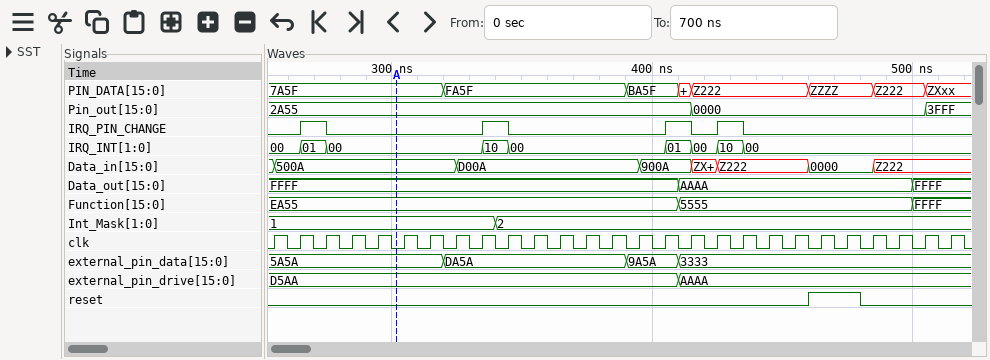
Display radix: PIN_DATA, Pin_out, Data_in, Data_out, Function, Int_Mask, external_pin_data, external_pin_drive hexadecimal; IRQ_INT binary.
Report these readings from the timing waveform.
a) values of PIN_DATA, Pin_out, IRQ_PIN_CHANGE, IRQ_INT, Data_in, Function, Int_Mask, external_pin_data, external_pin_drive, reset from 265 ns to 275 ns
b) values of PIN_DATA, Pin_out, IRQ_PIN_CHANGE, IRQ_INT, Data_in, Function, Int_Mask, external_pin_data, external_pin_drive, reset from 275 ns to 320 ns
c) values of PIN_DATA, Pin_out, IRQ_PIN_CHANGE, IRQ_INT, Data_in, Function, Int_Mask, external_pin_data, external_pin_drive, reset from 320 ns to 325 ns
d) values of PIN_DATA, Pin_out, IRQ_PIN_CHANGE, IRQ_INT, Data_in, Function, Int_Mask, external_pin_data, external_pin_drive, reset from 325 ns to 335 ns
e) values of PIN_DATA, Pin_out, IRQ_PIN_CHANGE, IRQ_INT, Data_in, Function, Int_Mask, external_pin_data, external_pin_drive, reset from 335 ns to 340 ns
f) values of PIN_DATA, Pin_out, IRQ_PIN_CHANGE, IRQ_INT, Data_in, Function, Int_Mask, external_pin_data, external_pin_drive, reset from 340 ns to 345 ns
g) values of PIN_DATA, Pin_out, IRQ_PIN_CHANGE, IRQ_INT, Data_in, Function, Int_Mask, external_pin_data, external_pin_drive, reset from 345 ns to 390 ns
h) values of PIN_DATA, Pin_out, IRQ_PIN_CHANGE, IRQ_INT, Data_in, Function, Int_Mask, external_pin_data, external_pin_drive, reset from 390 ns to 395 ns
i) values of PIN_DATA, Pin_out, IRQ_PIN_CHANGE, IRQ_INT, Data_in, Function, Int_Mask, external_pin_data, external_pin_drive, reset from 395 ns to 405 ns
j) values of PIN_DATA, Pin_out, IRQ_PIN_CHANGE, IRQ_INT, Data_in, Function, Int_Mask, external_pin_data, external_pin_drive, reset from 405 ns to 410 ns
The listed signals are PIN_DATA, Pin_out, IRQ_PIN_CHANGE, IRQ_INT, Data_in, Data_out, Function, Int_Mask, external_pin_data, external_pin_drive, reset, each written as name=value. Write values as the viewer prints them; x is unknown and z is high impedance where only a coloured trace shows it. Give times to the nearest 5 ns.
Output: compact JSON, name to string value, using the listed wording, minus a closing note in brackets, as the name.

{"values of PIN_DATA, Pin_out, IRQ_PIN_CHANGE, IRQ_INT, Data_in, Function, Int_Mask, external_pin_data, external_pin_drive, reset from 265 ns to 275 ns": "PIN_DATA=7A5F, Pin_out=2A55, IRQ_PIN_CHANGE=1, IRQ_INT=01, Data_in=500A, Function=EA55, Int_Mask=1, external_pin_data=5A5A, external_pin_drive=D5AA, reset=0", "values of PIN_DATA, Pin_out, IRQ_PIN_CHANGE, IRQ_INT, Data_in, Function, Int_Mask, external_pin_data, external_pin_drive, reset from 275 ns to 320 ns": "PIN_DATA=7A5F, Pin_out=2A55, IRQ_PIN_CHANGE=0, IRQ_INT=00, Data_in=500A, Function=EA55, Int_Mask=1, external_pin_data=5A5A, external_pin_drive=D5AA, reset=0", "values of PIN_DATA, Pin_out, IRQ_PIN_CHANGE, IRQ_INT, Data_in, Function, Int_Mask, external_pin_data, external_pin_drive, reset from 320 ns to 325 ns": "PIN_DATA=FA5F, Pin_out=2A55, IRQ_PIN_CHANGE=0, IRQ_INT=00, Data_in=500A, Function=EA55, Int_Mask=1, external_pin_data=DA5A, external_pin_drive=D5AA, reset=0", "values of PIN_DATA, Pin_out, IRQ_PIN_CHANGE, IRQ_INT, Data_in, Function, Int_Mask, external_pin_data, external_pin_drive, reset from 325 ns to 335 ns": "PIN_DATA=FA5F, Pin_out=2A55, IRQ_PIN_CHANGE=0, IRQ_INT=00, Data_in=D00A, Function=EA55, Int_Mask=1, external_pin_data=DA5A, external_pin_drive=D5AA, reset=0", "values of PIN_DATA, Pin_out, IRQ_PIN_CHANGE, IRQ_INT, Data_in, Function, Int_Mask, external_pin_data, external_pin_drive, reset from 335 ns to 340 ns": "PIN_DATA=FA5F, Pin_out=2A55, IRQ_PIN_CHANGE=1, IRQ_INT=10, Data_in=D00A, Function=EA55, Int_Mask=1, external_pin_data=DA5A, external_pin_drive=D5AA, reset=0", "values of PIN_DATA, Pin_out, IRQ_PIN_CHANGE, IRQ_INT, Data_in, Function, Int_Mask, external_pin_data, external_pin_drive, reset from 340 ns to 345 ns": "PIN_DATA=FA5F, Pin_out=2A55, IRQ_PIN_CHANGE=1, IRQ_INT=10, Data_in=D00A, Function=EA55, Int_Mask=2, external_pin_data=DA5A, external_pin_drive=D5AA, reset=0", "values of PIN_DATA, Pin_out, IRQ_PIN_CHANGE, IRQ_INT, Data_in, Function, Int_Mask, external_pin_data, external_pin_drive, reset from 345 ns to 390 ns": "PIN_DATA=FA5F, Pin_out=2A55, IRQ_PIN_CHANGE=0, IRQ_INT=00, Data_in=D00A, Function=EA55, Int_Mask=2, external_pin_data=DA5A, external_pin_drive=D5AA, reset=0", "values of PIN_DATA, Pin_out, IRQ_PIN_CHANGE, IRQ_INT, Data_in, Function, Int_Mask, external_pin_data, external_pin_drive, reset from 390 ns to 395 ns": "PIN_DATA=BA5F, Pin_out=2A55, IRQ_PIN_CHANGE=0, IRQ_INT=00, Data_in=D00A, Function=EA55, Int_Mask=2, external_pin_data=9A5A, external_pin_drive=D5AA, reset=0", "values of PIN_DATA, Pin_out, IRQ_PIN_CHANGE, IRQ_INT, Data_in, Function, Int_Mask, external_pin_data, external_pin_drive, reset from 395 ns to 405 ns": "PIN_DATA=BA5F, Pin_out=2A55, IRQ_PIN_CHANGE=0, IRQ_INT=00, Data_in=900A, Function=EA55, Int_Mask=2, external_pin_data=9A5A, external_pin_drive=D5AA, reset=0", "values of PIN_DATA, Pin_out, IRQ_PIN_CHANGE, IRQ_INT, Data_in, Function, Int_Mask, external_pin_data, external_pin_drive, reset from 405 ns to 410 ns": "PIN_DATA=BA5F, Pin_out=2A55, IRQ_PIN_CHANGE=1, IRQ_INT=01, Data_in=900A, Function=EA55, Int_Mask=2, external_pin_data=9A5A, external_pin_drive=D5AA, reset=0"}
